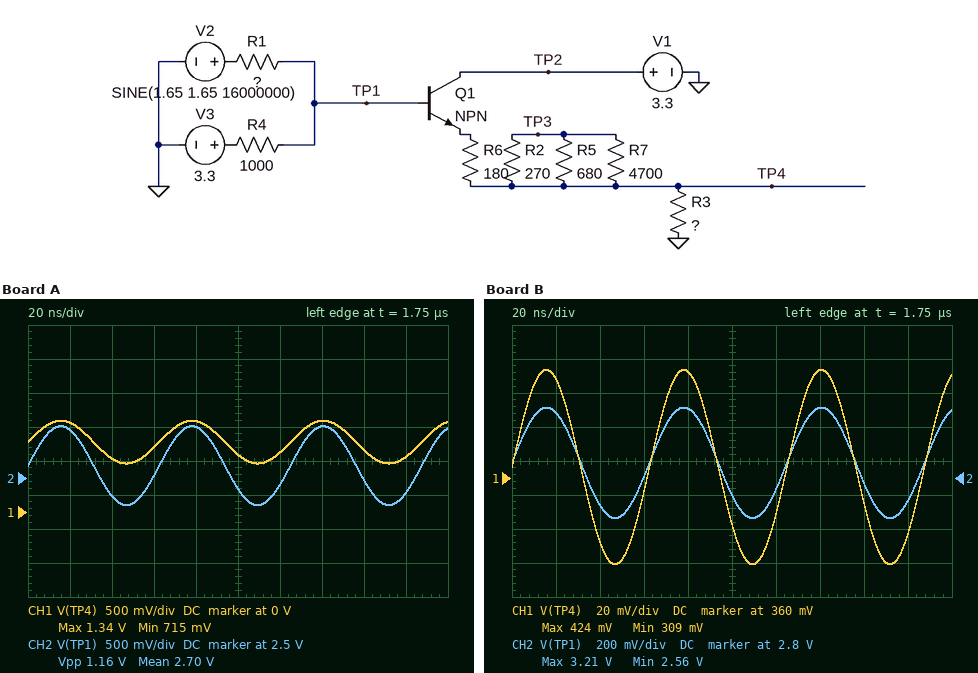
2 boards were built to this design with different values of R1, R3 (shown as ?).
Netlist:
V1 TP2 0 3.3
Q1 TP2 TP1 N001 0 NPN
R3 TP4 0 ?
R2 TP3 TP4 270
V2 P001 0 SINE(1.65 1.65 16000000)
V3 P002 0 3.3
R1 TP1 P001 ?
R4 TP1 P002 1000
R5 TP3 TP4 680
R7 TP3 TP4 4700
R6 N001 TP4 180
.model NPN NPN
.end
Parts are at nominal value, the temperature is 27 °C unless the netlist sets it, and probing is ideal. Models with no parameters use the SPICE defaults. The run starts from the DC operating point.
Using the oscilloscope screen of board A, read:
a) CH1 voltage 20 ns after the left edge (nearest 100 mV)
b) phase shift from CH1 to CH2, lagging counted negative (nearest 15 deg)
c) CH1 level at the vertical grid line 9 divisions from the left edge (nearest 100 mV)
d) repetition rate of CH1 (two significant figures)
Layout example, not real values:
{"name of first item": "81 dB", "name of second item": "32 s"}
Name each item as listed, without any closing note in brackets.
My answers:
{"CH1 voltage 20 ns after the left edge": "1.3 V", "phase shift from CH1 to CH2, lagging counted negative": "0 deg", "CH1 level at the vertical grid line 9 divisions from the left edge": "800 mV", "repetition rate of CH1": "16 MHz"}
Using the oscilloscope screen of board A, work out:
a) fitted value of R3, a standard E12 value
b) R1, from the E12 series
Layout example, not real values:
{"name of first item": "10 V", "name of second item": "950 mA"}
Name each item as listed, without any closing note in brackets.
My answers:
{"fitted value of R3, a standard E12 value": "220 Ω", "R1, from the E12 series": "1.8 kΩ"}
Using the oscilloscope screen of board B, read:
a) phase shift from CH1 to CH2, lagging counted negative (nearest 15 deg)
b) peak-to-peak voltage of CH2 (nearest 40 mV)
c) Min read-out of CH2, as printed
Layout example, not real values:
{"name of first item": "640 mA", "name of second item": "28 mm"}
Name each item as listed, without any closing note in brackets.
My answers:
{"phase shift from CH1 to CH2, lagging counted negative": "0 deg", "peak-to-peak voltage of CH2": "640 mV", "Min read-out of CH2, as printed": "2.56 V"}
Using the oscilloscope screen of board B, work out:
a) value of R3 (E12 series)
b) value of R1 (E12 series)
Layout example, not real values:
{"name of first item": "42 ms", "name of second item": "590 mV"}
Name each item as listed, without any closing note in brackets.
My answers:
{"value of R3": "39 Ω", "value of R1": "3.9 kΩ"}
